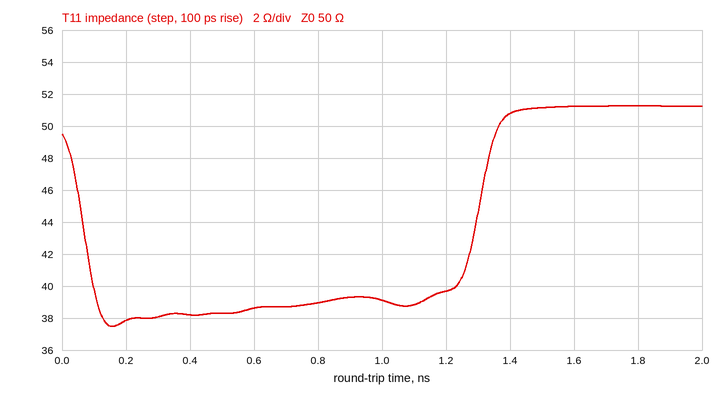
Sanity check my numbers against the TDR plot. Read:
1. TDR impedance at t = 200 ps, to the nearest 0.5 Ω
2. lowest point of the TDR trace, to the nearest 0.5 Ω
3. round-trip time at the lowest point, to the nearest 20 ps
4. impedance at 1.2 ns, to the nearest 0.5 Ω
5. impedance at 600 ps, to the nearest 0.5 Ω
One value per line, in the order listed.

38.0 Ω
37.5 Ω
160 ps
39.5 Ω
38.5 Ω
